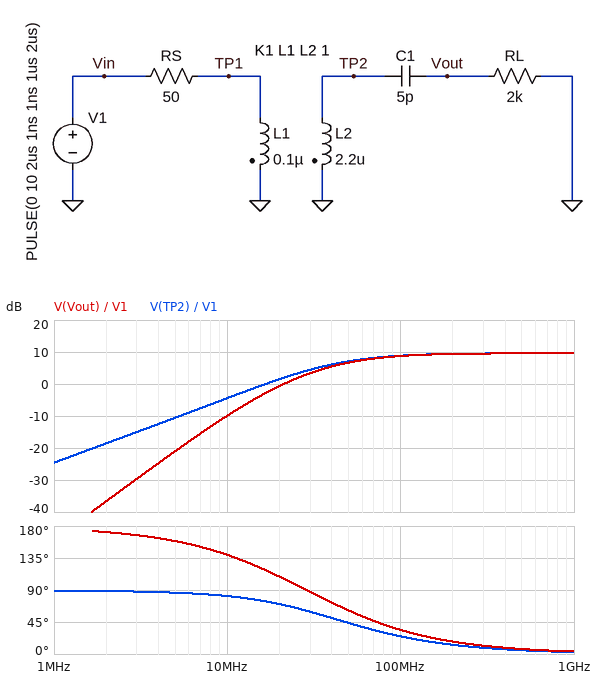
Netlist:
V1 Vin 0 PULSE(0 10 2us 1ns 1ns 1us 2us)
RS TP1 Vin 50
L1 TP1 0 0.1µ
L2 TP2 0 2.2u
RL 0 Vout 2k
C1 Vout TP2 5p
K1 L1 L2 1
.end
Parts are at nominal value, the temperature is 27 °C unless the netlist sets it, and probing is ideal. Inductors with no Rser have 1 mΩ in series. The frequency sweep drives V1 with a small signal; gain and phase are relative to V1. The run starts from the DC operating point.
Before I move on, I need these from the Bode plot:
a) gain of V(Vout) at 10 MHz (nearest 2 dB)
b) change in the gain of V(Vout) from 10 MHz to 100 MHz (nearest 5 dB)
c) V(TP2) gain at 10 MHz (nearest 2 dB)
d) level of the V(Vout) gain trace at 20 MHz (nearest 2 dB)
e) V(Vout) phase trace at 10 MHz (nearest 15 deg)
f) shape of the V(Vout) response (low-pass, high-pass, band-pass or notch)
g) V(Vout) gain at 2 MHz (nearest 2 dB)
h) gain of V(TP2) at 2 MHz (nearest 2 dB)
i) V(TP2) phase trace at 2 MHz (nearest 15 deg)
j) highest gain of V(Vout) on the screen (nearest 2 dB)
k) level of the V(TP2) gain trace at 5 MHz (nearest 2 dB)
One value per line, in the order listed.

-10 dB
20 dB
-4 dB
0 dB
135 deg
high-pass
-36 dB
-18 dB
90 deg
10 dB
-10 dB
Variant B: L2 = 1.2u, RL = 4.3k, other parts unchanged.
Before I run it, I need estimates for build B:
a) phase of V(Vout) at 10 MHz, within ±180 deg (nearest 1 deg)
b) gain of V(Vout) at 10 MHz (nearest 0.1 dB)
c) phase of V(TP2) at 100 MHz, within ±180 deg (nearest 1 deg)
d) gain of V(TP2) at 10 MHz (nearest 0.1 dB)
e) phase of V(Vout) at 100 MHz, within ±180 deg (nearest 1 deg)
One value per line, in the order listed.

119 deg
-9.1 dB
35 deg
-7.2 dB
39 deg
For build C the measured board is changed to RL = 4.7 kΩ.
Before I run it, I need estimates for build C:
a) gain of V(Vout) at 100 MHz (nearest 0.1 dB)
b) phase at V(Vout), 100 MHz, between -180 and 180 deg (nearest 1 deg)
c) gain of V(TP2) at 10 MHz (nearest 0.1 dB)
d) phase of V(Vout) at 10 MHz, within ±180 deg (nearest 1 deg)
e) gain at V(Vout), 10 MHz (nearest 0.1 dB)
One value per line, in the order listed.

10.1 dB
36 deg
-4.6 dB
116 deg
-6.2 dB
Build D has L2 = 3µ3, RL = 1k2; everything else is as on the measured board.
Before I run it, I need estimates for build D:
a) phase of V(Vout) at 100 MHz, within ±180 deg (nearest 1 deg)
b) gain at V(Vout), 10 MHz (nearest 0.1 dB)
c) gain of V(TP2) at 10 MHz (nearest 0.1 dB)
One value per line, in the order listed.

26 deg
-11.5 dB
-2.4 dB
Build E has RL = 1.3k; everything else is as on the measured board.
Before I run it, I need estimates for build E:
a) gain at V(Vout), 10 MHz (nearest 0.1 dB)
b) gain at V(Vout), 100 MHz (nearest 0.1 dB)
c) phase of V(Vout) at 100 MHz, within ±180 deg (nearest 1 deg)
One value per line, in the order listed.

-12.8 dB
7.6 dB
32 deg
